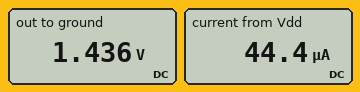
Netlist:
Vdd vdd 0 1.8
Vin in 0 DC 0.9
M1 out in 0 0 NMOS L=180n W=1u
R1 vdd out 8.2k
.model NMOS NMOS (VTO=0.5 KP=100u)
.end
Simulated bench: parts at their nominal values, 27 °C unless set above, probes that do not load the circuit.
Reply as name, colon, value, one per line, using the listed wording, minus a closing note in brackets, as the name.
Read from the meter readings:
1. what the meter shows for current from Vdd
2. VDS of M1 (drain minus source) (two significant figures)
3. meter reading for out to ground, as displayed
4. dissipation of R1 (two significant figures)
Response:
what the meter shows for current from Vdd: 44.4 µA
VDS of M1 (drain minus source): 1.4 V
meter reading for out to ground, as displayed: 1.436 V
dissipation of R1: 16 µW
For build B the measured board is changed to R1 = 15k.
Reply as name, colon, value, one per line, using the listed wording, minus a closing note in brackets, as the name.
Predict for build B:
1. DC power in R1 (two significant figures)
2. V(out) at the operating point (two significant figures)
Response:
DC power in R1: 30 µW
V(out) at the operating point: 1.1 V
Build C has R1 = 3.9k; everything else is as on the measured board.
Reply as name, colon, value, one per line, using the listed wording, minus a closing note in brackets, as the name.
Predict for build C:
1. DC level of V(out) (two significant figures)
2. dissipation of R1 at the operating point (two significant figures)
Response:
DC level of V(out): 1.6 V
dissipation of R1 at the operating point: 7.7 µW
